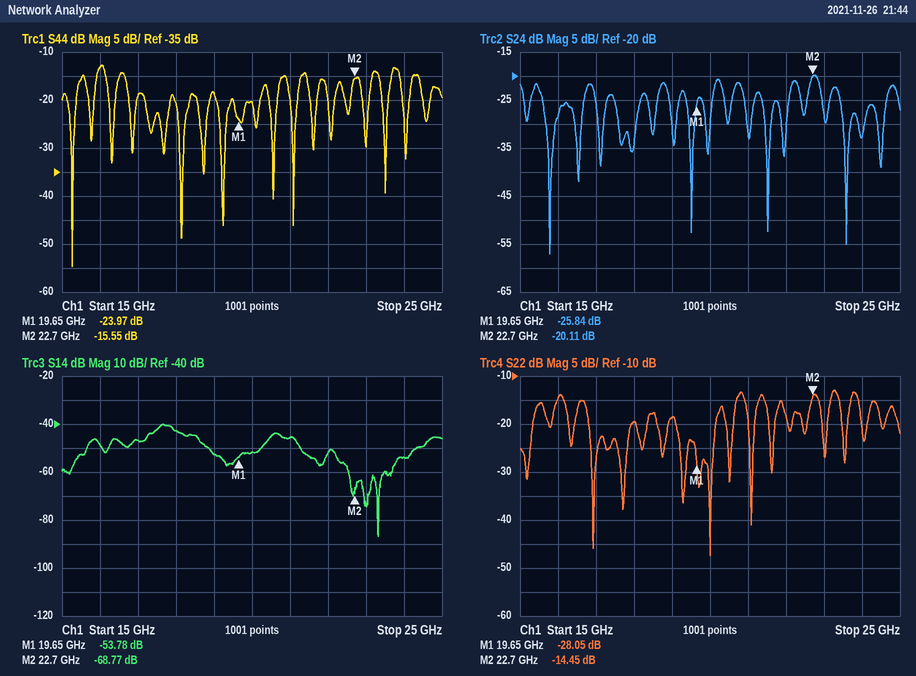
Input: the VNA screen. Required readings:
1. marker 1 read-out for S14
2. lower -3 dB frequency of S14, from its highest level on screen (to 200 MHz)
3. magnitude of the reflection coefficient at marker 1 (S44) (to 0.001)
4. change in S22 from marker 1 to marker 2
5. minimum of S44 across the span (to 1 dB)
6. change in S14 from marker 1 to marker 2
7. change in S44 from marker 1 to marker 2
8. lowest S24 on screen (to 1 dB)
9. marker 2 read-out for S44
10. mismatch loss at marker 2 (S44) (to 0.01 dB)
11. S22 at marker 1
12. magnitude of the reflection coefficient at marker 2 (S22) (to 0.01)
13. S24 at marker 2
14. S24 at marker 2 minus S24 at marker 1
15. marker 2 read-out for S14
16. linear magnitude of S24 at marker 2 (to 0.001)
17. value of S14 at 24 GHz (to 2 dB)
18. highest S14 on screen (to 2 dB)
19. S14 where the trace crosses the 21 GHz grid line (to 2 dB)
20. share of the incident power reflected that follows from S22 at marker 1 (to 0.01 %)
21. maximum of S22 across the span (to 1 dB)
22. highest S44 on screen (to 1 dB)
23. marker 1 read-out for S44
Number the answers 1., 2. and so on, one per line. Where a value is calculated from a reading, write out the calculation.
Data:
1. -53.78 dB
2. 17.4 GHz
3. 10^(-23.97/20) ≈ 0.063
4. -14.45 − (-28.05) = 13.60 dB
5. -55 dB
6. -68.77 − (-53.78) = -14.99 dB
7. -15.55 − (-23.97) = 8.42 dB
8. -57 dB
9. -15.55 dB
10. −10 log10(1 − 10^(-15.55/10)) ≈ 0.12 dB
11. -28.05 dB
12. 10^(-14.45/20) ≈ 0.19
13. -20.11 dB
14. -20.11 − (-25.84) = 5.73 dB
15. -68.77 dB
16. 10^(-20.11/20) ≈ 0.099
17. -54 dB
18. -40 dB
19. -46 dB
20. 10^(-28.05/10) ≈ 0.16 %
21. -13 dB
22. -13 dB
23. -23.97 dB
